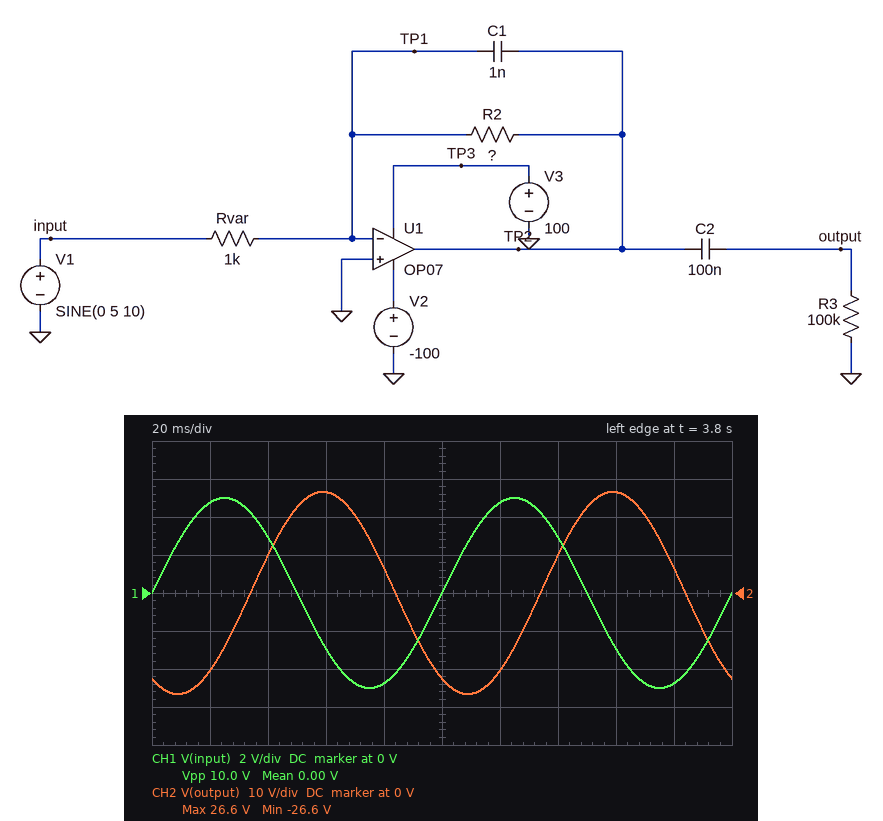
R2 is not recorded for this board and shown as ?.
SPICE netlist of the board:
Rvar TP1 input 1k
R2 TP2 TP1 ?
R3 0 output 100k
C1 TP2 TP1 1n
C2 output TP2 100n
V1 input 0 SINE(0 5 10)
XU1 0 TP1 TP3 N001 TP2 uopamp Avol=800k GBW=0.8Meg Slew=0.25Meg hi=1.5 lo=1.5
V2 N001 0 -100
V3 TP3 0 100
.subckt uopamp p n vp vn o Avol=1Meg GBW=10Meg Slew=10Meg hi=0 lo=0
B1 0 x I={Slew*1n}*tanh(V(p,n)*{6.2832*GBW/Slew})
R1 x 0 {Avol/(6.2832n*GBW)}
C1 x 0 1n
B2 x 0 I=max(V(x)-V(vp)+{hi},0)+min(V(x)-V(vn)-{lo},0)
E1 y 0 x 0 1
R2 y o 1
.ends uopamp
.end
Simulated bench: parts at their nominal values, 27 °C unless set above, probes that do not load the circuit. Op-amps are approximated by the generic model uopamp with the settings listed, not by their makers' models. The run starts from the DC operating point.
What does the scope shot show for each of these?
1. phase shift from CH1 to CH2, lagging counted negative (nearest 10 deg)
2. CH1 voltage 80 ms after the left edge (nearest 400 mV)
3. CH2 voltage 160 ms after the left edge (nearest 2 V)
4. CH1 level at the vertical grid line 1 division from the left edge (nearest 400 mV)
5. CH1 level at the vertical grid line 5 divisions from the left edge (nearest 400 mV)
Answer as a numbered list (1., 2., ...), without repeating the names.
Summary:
1. -120 deg
2. -4.8 V
3. 26 V
4. 4.8 V
5. 0 V
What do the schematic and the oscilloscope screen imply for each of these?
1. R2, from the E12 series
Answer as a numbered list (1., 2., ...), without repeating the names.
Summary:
1. 10 kΩ
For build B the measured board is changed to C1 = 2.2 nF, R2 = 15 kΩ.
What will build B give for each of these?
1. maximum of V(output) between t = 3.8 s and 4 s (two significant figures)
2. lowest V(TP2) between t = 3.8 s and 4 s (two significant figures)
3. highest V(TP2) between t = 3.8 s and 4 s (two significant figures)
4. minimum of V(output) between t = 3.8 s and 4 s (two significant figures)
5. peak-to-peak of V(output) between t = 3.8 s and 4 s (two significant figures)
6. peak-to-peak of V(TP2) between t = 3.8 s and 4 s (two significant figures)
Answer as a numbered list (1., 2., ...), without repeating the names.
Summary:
1. 40 V
2. -75 V
3. 75 V
4. -40 V
5. 80 V
6. 150 V
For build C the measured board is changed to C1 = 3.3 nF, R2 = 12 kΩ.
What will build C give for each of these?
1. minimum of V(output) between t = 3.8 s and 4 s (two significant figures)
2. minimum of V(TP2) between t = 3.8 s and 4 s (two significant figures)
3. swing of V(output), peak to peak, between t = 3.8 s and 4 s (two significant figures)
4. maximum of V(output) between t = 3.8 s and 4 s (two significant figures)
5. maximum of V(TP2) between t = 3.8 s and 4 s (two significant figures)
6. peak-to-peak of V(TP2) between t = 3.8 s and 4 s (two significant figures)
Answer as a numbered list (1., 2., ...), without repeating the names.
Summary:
1. -32 V
2. -60 V
3. 64 V
4. 32 V
5. 60 V
6. 120 V
